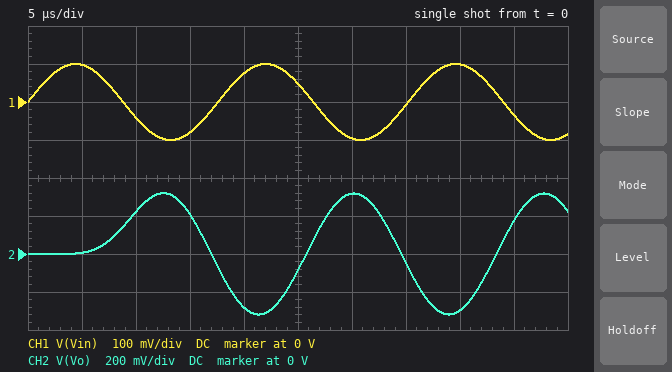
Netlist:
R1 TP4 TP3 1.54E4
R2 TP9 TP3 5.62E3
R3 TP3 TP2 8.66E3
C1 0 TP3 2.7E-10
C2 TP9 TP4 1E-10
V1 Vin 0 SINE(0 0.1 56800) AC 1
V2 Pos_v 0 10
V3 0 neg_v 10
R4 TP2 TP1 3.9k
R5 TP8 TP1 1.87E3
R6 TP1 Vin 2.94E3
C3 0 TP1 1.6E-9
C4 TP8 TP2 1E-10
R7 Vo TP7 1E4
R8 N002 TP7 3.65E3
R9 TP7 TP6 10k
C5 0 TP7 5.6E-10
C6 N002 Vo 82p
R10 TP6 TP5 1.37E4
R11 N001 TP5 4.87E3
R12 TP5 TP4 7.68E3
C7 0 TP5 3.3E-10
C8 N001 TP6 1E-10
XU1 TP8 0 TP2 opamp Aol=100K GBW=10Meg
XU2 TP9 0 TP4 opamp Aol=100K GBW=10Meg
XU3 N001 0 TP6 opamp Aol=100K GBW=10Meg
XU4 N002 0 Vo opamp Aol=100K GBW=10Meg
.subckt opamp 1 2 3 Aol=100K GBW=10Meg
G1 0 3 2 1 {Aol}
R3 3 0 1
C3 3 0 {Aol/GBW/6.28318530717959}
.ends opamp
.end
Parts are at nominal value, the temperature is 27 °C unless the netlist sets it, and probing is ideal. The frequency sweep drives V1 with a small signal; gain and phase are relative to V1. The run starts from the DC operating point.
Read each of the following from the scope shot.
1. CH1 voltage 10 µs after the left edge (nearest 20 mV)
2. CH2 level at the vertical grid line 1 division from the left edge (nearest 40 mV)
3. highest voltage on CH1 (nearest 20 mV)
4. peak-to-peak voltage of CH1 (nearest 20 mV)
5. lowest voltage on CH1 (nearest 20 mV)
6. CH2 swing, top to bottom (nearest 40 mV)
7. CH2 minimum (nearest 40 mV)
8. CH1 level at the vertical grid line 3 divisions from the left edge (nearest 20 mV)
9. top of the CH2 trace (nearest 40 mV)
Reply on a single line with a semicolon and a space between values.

-40 mV; 0 V; 100 mV; 200 mV; -100 mV; 640 mV; -320 mV; -80 mV; 320 mV
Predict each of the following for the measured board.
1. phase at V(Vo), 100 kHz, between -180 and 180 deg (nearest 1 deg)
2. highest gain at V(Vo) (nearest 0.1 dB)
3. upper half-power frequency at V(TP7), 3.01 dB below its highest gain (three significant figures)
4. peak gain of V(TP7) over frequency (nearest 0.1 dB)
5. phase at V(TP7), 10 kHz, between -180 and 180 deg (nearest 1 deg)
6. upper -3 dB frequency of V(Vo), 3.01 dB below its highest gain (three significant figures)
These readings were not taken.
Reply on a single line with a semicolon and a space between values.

64 deg; 12.5 dB; 118 kHz; -8.2 dB; -120 deg; 63.7 kHz
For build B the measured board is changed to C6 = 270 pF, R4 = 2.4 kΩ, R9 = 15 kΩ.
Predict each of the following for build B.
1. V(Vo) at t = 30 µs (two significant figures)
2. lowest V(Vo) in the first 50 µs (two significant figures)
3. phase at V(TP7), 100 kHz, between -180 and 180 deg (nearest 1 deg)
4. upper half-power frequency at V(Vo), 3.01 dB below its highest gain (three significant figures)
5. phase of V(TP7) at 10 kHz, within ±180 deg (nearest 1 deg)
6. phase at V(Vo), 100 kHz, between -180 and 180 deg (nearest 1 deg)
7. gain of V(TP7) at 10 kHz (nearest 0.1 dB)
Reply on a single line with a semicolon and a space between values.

54 mV; -74 mV; -49 deg; 35.2 kHz; -129 deg; 40 deg; -19.5 dB
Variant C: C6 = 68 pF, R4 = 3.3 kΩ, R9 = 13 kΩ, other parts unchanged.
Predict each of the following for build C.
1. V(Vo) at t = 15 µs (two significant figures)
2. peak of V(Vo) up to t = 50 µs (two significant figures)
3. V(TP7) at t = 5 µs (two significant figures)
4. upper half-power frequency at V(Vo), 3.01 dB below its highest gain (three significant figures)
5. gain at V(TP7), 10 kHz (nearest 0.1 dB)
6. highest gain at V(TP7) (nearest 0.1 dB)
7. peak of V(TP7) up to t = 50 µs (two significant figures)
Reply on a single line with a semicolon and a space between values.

110 mV; 210 mV; -2.0 mV; 65.8 kHz; -26.9 dB; -13.0 dB; 20 mV
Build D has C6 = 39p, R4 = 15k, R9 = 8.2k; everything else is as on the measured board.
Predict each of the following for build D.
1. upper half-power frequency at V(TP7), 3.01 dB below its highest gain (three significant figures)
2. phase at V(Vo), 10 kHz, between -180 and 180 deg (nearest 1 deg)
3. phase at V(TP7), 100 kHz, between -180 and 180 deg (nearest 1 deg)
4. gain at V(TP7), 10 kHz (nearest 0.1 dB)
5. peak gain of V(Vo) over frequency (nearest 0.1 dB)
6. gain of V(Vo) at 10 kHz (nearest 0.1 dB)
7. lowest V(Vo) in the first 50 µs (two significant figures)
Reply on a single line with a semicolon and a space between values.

84.7 kHz; -34 deg; -60 deg; -14.2 dB; 25.9 dB; 25.8 dB; -1.3 V
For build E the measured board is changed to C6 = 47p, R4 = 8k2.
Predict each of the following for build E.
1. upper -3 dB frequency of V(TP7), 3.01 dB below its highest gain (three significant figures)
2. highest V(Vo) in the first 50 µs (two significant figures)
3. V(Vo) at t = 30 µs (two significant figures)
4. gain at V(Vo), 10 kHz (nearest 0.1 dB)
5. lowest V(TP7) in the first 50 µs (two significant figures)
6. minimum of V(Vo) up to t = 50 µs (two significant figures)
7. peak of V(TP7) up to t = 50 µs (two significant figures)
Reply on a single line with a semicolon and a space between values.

106 kHz; 700 mV; 690 mV; 18.9 dB; -47 mV; -700 mV; 47 mV
